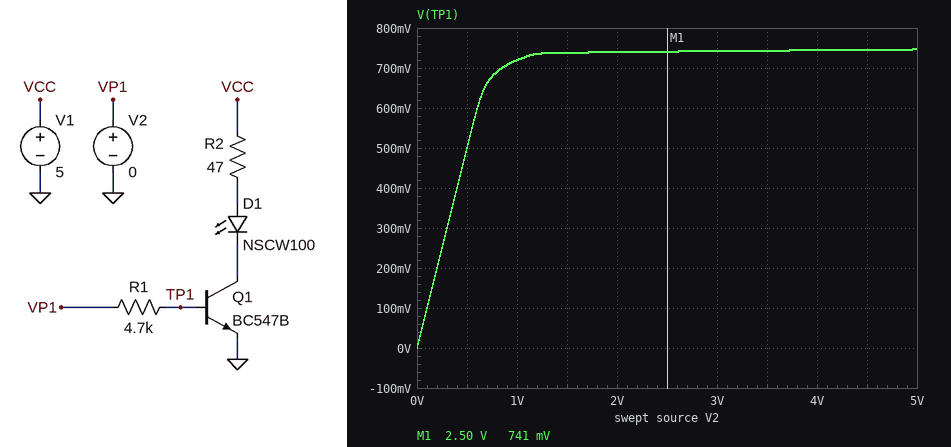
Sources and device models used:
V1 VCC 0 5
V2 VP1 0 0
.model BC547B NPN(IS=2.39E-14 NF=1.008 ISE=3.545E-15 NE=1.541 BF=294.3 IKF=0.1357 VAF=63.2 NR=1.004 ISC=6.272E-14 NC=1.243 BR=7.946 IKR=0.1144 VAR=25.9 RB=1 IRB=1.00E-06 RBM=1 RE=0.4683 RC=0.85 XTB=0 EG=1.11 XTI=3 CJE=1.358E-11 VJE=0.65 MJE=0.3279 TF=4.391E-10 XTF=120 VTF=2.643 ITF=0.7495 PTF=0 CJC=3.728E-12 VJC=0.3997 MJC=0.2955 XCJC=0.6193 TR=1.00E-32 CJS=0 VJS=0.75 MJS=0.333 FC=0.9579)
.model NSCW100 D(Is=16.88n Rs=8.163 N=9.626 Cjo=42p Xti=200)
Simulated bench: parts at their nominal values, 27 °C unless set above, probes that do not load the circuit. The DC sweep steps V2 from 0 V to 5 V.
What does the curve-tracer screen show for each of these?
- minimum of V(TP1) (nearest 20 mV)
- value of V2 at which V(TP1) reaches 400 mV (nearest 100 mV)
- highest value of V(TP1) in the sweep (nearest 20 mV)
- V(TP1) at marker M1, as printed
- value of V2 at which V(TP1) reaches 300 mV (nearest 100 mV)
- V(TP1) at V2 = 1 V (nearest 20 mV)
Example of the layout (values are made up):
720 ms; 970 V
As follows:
0 V; 400 mV; 740 mV; 741 mV; 300 mV; 720 mV
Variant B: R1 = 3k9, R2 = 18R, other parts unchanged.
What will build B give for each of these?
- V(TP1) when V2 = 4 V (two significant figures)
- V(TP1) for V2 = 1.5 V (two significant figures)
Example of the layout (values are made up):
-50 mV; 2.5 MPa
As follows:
770 mV; 760 mV
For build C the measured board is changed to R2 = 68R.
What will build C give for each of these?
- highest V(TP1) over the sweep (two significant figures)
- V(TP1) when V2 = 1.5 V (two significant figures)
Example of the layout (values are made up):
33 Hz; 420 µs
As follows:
740 mV; 730 mV
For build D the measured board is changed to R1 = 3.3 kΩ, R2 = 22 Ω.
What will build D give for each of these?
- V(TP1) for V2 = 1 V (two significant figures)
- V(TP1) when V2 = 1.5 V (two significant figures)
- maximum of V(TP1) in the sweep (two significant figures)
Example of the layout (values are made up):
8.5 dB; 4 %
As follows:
730 mV; 760 mV; 770 mV
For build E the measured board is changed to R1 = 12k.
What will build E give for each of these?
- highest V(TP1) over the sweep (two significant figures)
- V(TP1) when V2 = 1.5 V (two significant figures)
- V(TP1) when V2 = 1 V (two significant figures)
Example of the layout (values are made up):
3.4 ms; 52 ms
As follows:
740 mV; 720 mV; 690 mV
